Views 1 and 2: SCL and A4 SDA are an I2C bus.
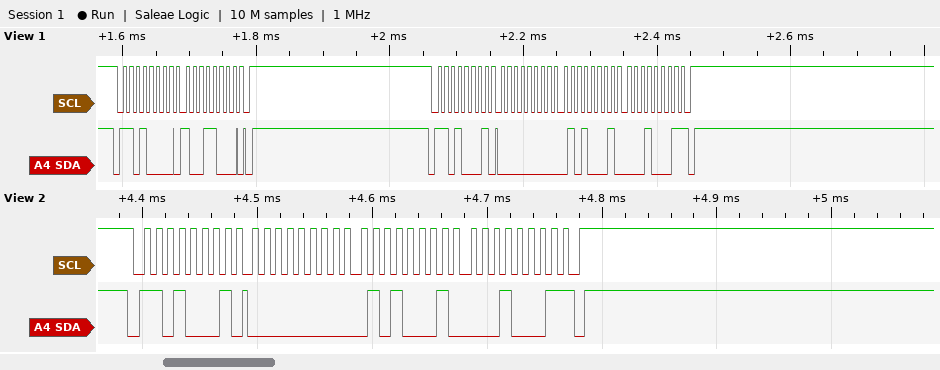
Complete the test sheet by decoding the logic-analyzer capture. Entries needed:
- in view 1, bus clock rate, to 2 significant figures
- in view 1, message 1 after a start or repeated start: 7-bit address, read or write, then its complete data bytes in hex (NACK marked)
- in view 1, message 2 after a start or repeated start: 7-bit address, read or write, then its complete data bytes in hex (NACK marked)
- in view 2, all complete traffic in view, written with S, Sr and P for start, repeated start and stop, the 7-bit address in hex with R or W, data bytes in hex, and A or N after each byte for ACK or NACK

100 kHz
0x68 write: 98
0x68 read: 00 51 11 NACK
S 68R A 00 A 51 A 11 N P
